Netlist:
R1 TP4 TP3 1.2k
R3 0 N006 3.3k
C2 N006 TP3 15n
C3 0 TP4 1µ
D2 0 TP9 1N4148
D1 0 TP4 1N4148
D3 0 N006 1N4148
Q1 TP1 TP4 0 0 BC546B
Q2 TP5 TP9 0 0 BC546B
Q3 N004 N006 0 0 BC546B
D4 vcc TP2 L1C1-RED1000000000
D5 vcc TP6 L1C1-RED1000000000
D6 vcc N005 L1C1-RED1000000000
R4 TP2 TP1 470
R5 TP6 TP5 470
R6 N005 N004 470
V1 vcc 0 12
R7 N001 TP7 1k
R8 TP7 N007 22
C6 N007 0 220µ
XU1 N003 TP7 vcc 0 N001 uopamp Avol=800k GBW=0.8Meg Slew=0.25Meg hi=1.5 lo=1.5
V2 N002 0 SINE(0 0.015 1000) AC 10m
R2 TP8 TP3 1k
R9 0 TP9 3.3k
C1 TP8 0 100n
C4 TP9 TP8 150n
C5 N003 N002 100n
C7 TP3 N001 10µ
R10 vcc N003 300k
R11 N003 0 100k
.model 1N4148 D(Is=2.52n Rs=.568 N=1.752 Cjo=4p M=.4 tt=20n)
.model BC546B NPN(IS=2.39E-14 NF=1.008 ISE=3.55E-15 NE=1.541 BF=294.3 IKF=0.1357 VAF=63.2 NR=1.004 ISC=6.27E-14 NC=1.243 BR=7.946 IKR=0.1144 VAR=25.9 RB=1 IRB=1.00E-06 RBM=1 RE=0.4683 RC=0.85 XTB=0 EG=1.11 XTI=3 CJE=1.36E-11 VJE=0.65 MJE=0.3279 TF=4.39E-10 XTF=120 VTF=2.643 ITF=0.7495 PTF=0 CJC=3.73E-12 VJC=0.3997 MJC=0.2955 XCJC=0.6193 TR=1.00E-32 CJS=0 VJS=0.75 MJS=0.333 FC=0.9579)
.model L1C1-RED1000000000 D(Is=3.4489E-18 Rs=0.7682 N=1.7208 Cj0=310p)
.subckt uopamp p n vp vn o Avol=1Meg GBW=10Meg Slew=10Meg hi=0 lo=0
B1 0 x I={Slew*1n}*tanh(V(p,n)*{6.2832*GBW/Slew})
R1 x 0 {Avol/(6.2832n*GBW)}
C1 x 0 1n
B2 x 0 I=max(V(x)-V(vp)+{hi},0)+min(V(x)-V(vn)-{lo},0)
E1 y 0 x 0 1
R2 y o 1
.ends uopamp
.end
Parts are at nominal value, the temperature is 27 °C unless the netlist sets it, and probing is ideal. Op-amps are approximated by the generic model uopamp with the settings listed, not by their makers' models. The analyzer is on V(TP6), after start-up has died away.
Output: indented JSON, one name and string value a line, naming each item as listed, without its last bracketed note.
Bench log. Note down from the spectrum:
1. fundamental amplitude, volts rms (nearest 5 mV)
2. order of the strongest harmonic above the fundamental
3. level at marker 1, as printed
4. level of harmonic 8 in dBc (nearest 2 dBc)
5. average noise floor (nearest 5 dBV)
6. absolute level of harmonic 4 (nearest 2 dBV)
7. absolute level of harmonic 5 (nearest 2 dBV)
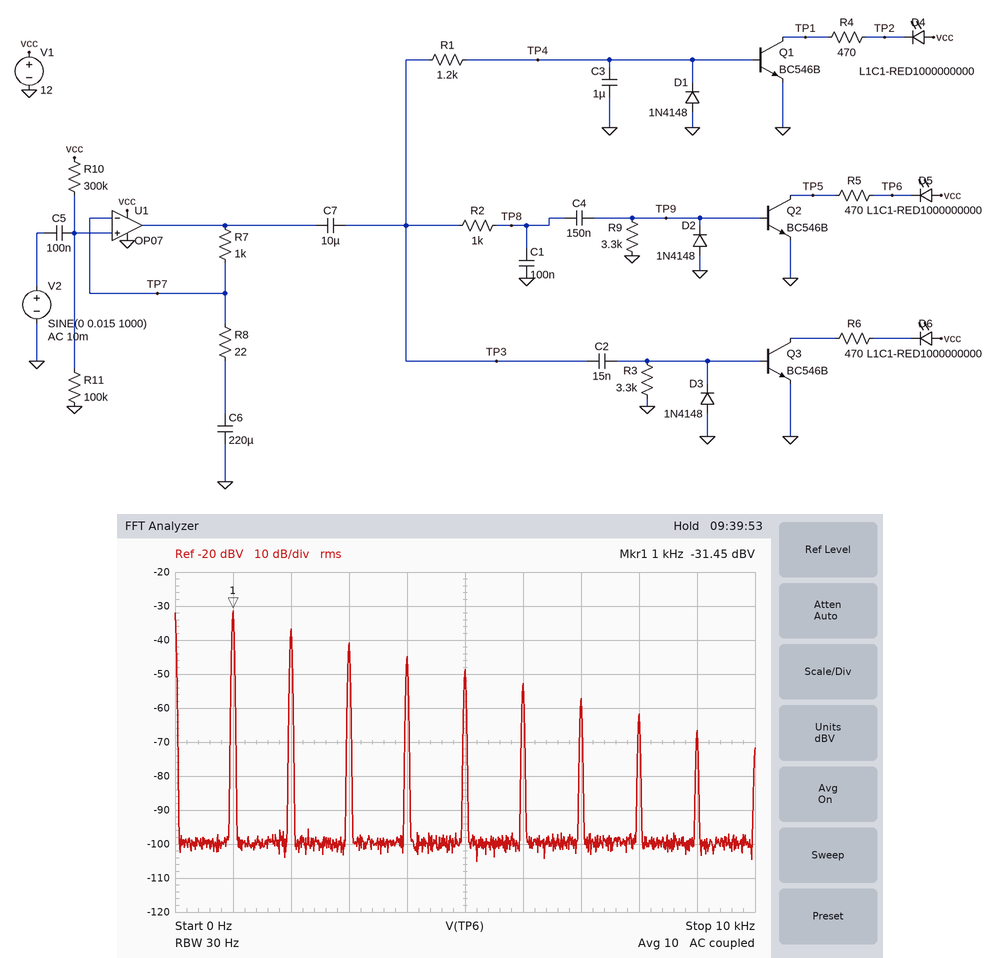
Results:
{
  "fundamental amplitude, volts rms": "25 mV",
  "order of the strongest harmonic above the fundamental": "2",
  "level at marker 1, as printed": "-31.45 dBV",
  "level of harmonic 8 in dBc": "-30 dBc",
  "average noise floor": "-100 dBV",
  "absolute level of harmonic 4": "-44 dBV",
  "absolute level of harmonic 5": "-48 dBV"
}
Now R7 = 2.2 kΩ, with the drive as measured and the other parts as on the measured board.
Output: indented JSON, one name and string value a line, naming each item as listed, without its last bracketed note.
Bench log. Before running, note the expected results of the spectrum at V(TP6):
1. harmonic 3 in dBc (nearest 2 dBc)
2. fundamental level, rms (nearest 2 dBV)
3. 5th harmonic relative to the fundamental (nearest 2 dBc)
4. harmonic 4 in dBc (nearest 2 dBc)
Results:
{
  "harmonic 3 in dBc": "-18 dBc",
  "fundamental level, rms": "-14 dBV",
  "5th harmonic relative to the fundamental": "-16 dBc",
  "harmonic 4 in dBc": "-16 dBc"
}
